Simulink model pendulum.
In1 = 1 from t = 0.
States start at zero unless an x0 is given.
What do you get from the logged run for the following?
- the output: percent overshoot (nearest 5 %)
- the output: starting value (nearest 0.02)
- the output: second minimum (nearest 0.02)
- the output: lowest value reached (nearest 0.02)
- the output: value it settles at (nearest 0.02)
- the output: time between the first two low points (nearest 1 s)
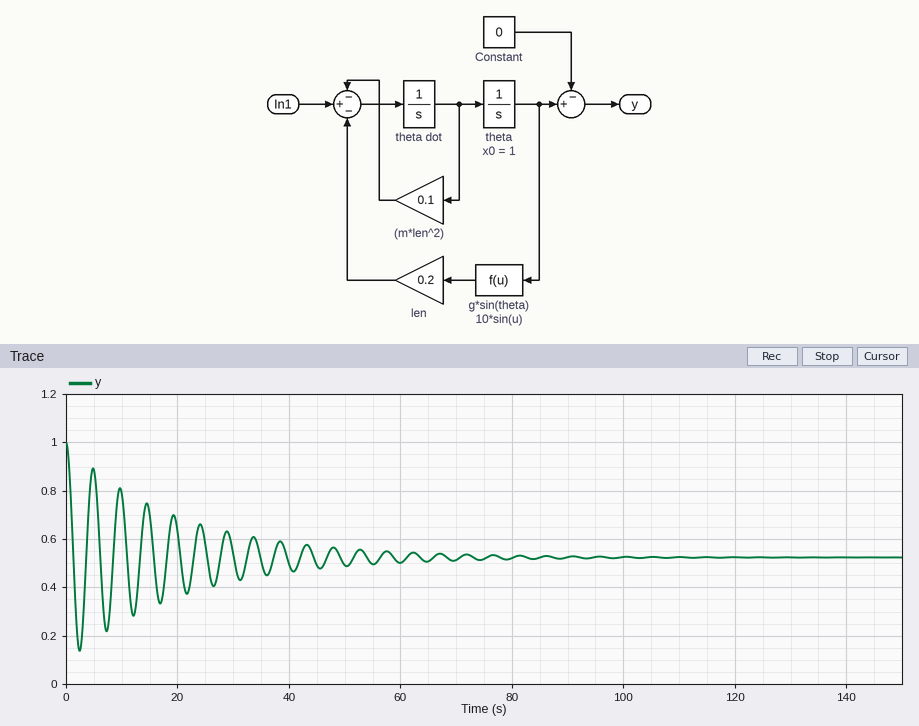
80 %
1.00
0.22
0.14
0.52
5 s
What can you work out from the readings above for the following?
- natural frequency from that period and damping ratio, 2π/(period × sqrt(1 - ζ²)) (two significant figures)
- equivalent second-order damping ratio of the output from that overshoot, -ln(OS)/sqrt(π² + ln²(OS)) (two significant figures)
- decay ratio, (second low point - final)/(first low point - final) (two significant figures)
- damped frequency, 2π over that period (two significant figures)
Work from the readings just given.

1.3 rad/s
0.071
0.79
1.3 rad/s
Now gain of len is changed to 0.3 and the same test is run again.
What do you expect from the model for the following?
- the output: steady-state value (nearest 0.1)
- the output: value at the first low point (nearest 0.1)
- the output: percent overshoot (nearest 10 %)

0.3
-0.2
80 %
